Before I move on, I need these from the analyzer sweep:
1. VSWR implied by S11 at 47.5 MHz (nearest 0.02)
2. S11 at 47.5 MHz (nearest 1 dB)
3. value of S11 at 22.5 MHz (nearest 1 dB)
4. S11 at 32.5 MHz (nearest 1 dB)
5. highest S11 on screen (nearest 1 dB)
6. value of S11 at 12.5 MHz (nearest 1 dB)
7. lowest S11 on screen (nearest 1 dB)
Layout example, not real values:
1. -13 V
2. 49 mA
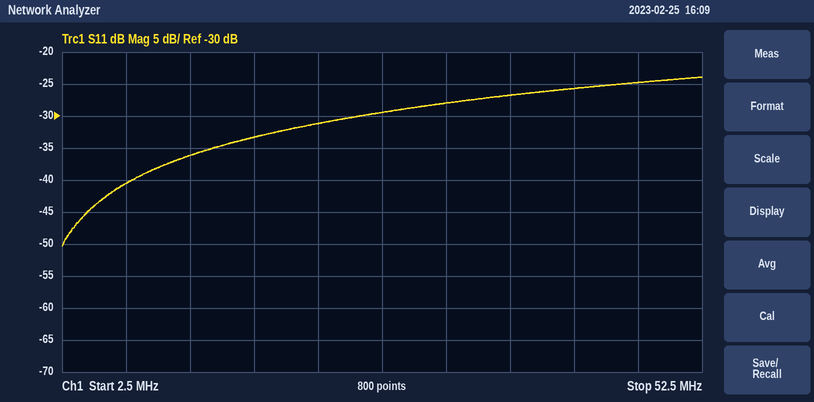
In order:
1. 1.12
2. -25 dB
3. -31 dB
4. -28 dB
5. -24 dB
6. -36 dB
7. -50 dB
